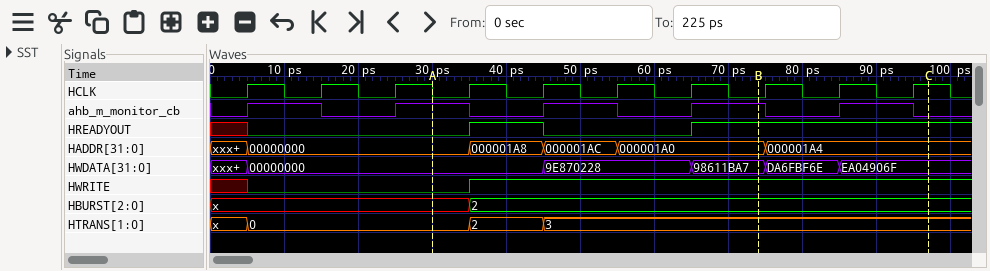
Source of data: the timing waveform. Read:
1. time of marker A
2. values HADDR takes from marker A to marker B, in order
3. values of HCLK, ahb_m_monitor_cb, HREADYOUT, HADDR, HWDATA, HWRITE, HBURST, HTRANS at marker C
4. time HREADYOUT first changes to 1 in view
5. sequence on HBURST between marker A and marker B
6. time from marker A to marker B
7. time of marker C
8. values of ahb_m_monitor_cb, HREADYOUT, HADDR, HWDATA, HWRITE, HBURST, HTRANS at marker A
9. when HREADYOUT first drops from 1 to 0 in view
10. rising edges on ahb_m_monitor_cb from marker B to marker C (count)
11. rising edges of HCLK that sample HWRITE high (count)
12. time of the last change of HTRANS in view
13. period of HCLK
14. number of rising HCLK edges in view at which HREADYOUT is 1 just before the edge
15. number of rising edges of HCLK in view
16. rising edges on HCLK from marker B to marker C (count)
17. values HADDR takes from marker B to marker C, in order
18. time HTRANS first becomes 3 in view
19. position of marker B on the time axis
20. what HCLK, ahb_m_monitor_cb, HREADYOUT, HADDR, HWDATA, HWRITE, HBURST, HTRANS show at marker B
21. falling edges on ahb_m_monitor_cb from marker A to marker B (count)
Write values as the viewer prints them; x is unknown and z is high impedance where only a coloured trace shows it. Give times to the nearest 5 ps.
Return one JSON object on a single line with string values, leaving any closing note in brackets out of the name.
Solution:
{"time of marker A": "30 ps", "values HADDR takes from marker A to marker B, in order": "00000000, 000001A8, 000001AC, 000001A0", "values of HCLK, ahb_m_monitor_cb, HREADYOUT, HADDR, HWDATA, HWRITE, HBURST, HTRANS at marker C": "HCLK=1, ahb_m_monitor_cb=0, HREADYOUT=1, HADDR=000001A4, HWDATA=EA04906F, HWRITE=1, HBURST=2, HTRANS=3", "time HREADYOUT first changes to 1 in view": "35 ps", "sequence on HBURST between marker A and marker B": "x, 2", "time from marker A to marker B": "45 ps", "time of marker C": "95 ps", "values of ahb_m_monitor_cb, HREADYOUT, HADDR, HWDATA, HWRITE, HBURST, HTRANS at marker A": "ahb_m_monitor_cb=1, HREADYOUT=0, HADDR=00000000, HWDATA=00000000, HWRITE=0, HBURST=x, HTRANS=0", "when HREADYOUT first drops from 1 to 0 in view": "45 ps", "rising edges on ahb_m_monitor_cb from marker B to marker C": "1", "rising edges of HCLK that sample HWRITE high": "6", "time of the last change of HTRANS in view": "45 ps", "period of HCLK": "10 ps", "number of rising HCLK edges in view at which HREADYOUT is 1 just before the edge": "4", "number of rising edges of HCLK in view": "10", "rising edges on HCLK from marker B to marker C": "3", "values HADDR takes from marker B to marker C, in order": "000001A0, 000001A4", "time HTRANS first becomes 3 in view": "45 ps", "position of marker B on the time axis": "75 ps", "what HCLK, ahb_m_monitor_cb, HREADYOUT, HADDR, HWDATA, HWRITE, HBURST, HTRANS show at marker B": "HCLK=0, ahb_m_monitor_cb=1, HREADYOUT=1, HADDR=000001A0, HWDATA=98611BA7, HWRITE=1, HBURST=2, HTRANS=3", "falling edges on ahb_m_monitor_cb from marker A to marker B": "2"}
